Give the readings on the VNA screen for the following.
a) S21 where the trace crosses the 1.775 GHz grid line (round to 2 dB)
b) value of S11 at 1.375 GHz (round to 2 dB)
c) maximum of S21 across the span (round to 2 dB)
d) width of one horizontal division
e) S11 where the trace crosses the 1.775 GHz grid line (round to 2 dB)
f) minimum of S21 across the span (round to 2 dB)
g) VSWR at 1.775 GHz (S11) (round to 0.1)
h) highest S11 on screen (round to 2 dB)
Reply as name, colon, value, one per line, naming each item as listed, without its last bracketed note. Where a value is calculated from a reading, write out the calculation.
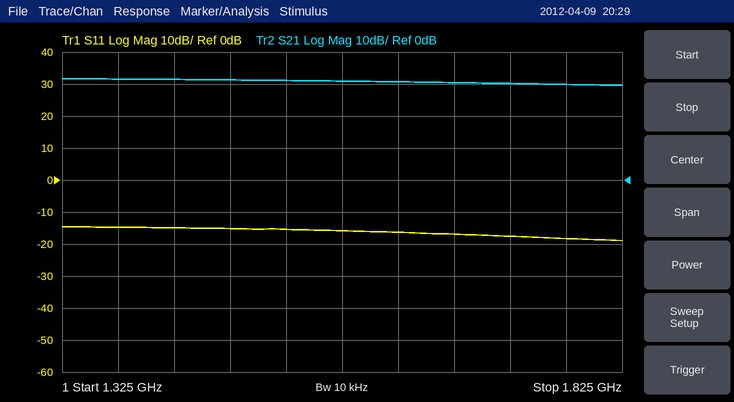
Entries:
S21 where the trace crosses the 1.775 GHz grid line: 30 dB
value of S11 at 1.375 GHz: -14 dB
maximum of S21 across the span: 32 dB
width of one horizontal division: 50 MHz
S11 where the trace crosses the 1.775 GHz grid line: -18 dB
minimum of S21 across the span: 30 dB
VSWR at 1.775 GHz (S11): |Γ| = 10^(-18/20) = 0.1259; VSWR = (1 + 0.1259)/(1 − 0.1259) ≈ 1.3
highest S11 on screen: -14 dB
